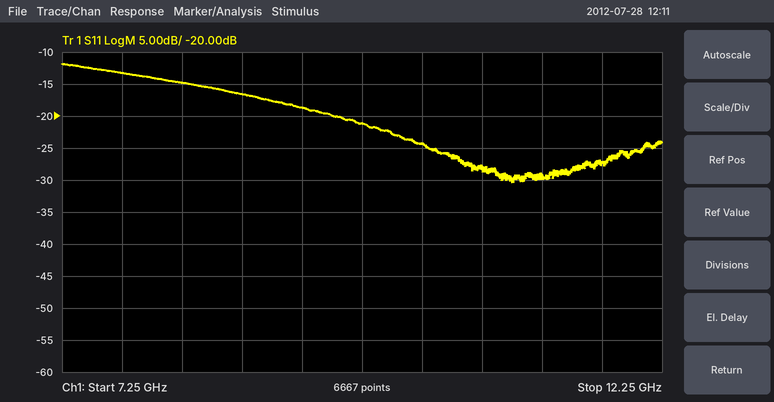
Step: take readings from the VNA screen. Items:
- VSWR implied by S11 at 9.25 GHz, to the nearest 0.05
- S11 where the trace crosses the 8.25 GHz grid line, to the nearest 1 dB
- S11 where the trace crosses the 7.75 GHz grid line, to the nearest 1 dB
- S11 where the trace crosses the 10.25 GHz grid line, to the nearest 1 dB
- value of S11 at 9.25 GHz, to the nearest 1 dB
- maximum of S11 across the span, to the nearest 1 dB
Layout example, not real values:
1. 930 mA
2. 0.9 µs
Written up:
1. 1.25
2. -15 dB
3. -13 dB
4. -24 dB
5. -19 dB
6. -12 dB
